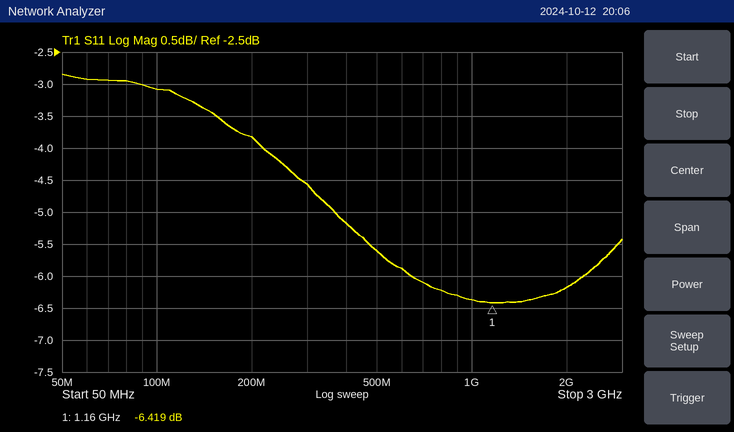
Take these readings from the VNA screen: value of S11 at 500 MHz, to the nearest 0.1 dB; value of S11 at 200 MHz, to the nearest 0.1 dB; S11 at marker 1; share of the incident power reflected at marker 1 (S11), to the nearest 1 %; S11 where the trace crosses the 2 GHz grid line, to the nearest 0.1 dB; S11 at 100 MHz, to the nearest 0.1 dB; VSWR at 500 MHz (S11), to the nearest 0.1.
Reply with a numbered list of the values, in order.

1. -5.6 dB
2. -3.8 dB
3. -6.419 dB
4. 23 %
5. -6.2 dB
6. -3.1 dB
7. 3.2
